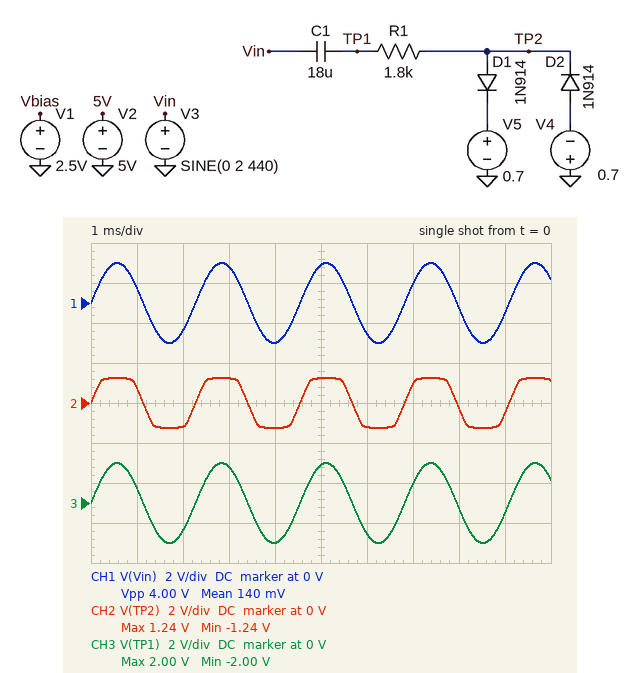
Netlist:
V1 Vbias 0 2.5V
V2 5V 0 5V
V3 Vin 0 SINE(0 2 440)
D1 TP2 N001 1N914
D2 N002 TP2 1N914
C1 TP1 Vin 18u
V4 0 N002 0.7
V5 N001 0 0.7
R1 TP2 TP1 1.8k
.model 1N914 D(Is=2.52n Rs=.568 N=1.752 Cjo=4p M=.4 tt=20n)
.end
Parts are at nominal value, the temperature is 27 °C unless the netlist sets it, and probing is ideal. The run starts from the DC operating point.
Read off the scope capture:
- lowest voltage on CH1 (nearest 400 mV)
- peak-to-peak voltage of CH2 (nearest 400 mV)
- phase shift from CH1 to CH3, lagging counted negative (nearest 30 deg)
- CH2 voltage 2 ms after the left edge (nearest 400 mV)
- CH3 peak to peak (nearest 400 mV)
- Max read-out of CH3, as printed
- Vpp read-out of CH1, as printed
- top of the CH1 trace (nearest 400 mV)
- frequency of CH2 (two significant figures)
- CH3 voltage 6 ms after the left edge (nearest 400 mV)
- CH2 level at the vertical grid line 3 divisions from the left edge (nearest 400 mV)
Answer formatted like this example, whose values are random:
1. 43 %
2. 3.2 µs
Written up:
1. -2.0 V
2. 2.4 V
3. 0 deg
4. -1.2 V
5. 4.0 V
6. 2.00 V
7. 4.00 V
8. 2.0 V
9. 440 Hz
10. -1.6 V
11. 1.2 V
